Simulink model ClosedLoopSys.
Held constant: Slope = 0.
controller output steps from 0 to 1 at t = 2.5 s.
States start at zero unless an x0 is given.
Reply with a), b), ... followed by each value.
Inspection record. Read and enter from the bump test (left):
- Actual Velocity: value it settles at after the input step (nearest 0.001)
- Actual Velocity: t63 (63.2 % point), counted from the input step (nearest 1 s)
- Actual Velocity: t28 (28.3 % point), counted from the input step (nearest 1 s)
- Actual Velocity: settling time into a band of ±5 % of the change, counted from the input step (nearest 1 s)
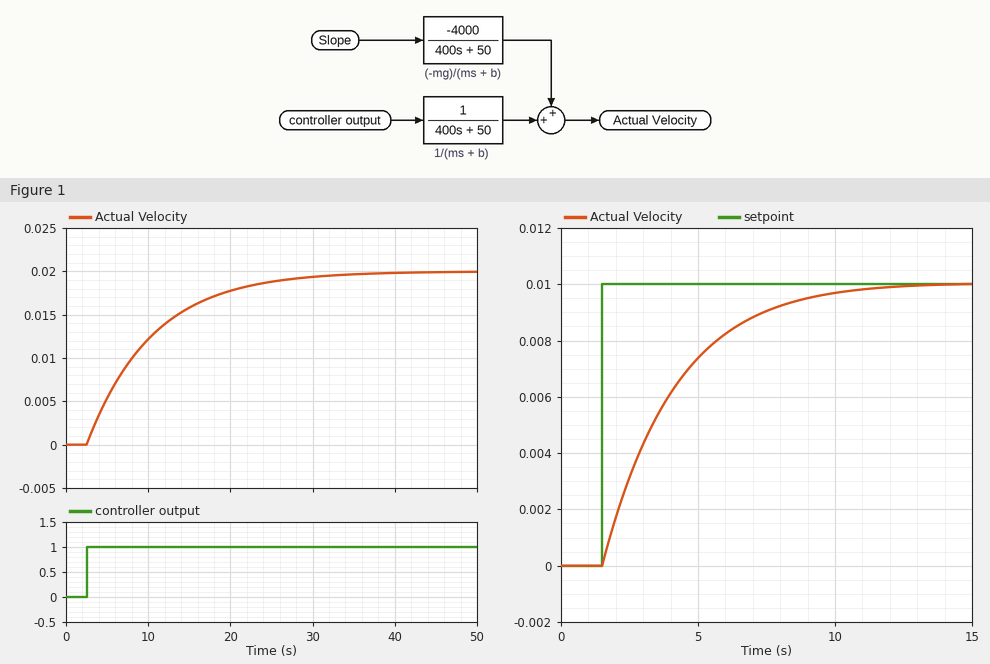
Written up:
a) 0.020
b) 8 s
c) 3 s
d) 24 s
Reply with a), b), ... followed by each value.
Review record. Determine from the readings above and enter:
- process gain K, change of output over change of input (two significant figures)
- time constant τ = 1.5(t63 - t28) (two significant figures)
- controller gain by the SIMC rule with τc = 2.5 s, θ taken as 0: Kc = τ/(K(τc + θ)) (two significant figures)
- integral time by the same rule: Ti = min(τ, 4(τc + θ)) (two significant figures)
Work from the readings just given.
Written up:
a) 0.020
b) 7.5 s
c) 150
d) 7.5 s
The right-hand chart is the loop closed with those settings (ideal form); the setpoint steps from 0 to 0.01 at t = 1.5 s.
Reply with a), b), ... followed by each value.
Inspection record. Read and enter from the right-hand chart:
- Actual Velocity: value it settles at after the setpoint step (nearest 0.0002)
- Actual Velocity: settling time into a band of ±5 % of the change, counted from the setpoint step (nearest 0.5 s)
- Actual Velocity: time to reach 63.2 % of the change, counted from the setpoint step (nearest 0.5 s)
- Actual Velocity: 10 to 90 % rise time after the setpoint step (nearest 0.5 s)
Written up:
a) 0.0100
b) 7.5 s
c) 2.5 s
d) 5.5 s
